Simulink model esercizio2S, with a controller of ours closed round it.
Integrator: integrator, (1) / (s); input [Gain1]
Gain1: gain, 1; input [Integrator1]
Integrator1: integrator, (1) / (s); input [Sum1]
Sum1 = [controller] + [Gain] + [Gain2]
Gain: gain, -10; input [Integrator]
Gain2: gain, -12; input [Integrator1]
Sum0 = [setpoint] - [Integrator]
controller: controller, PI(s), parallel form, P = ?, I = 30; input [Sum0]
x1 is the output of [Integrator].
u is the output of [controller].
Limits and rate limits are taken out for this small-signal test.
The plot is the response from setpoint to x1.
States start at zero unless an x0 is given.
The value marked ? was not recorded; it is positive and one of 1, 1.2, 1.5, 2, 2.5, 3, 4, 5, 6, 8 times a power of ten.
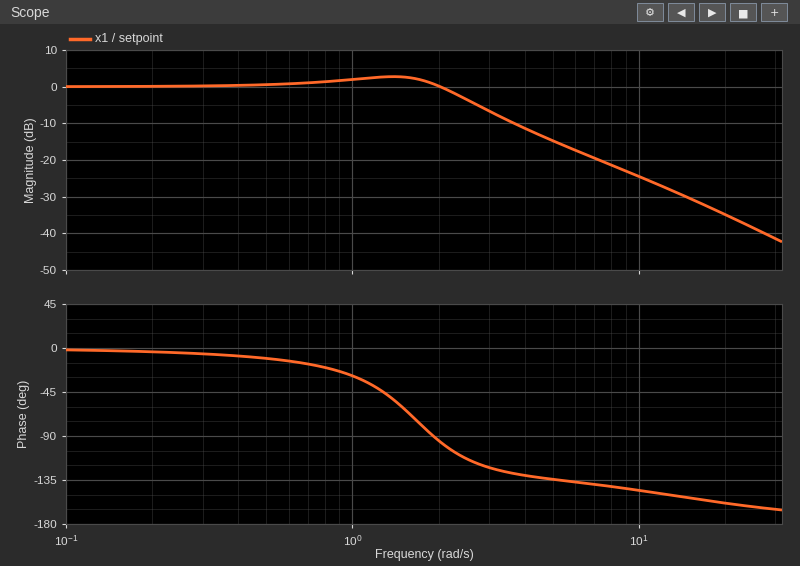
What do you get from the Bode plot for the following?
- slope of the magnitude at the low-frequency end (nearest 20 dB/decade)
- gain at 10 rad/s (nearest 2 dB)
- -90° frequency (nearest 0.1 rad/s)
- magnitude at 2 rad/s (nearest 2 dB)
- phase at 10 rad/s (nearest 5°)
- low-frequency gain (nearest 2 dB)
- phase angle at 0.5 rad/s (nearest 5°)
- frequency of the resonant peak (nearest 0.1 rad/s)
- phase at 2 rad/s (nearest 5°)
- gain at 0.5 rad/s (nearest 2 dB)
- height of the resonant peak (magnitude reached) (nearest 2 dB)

0 dB/decade
-24 dB
1.9 rad/s
0 dB
-145°
0 dB
-10°
1.4 rad/s
-95°
0 dB
2 dB
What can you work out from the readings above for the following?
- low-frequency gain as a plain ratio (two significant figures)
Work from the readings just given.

1.0
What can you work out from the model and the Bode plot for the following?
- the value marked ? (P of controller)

8
